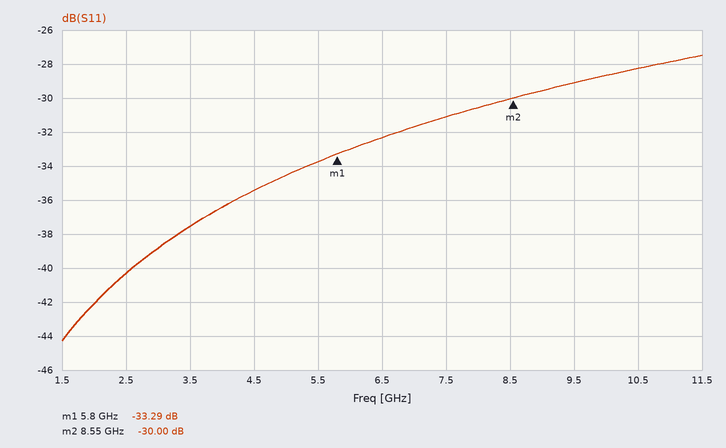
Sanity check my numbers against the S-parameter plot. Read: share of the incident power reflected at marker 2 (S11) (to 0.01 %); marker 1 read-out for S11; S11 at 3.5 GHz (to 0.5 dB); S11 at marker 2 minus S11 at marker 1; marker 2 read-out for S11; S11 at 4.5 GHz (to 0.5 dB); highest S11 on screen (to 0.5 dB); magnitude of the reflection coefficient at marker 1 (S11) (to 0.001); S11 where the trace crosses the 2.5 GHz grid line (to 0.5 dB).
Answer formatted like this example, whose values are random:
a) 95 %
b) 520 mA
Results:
a) 0.10 %
b) -33.29 dB
c) -37.5 dB
d) 3.29 dB
e) -30.00 dB
f) -35.5 dB
g) -27.5 dB
h) 0.022
i) -40.5 dB
